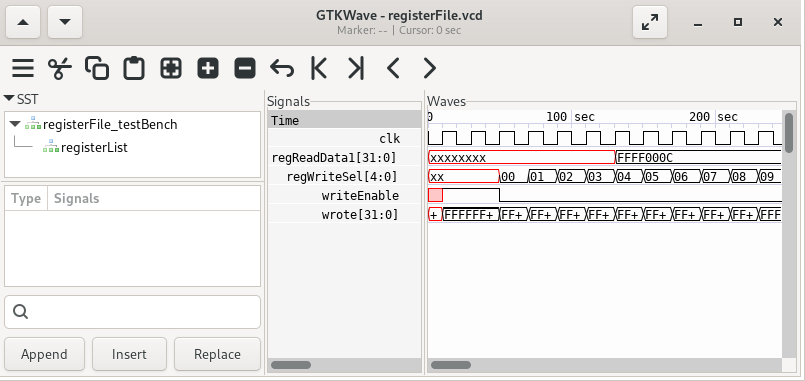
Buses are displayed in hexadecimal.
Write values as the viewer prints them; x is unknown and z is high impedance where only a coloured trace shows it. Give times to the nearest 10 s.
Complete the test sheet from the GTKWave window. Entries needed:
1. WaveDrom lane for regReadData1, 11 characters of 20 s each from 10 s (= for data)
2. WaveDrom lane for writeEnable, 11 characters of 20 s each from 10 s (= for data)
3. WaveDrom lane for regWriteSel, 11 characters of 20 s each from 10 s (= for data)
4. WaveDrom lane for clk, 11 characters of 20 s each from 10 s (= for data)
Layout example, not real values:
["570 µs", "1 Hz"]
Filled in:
["{name: 'regReadData1', wave: 'x.....=....', data: 'FFFF000C'}", "{name: 'writeEnable', wave: '1.0........'}", "{name: 'regWriteSel', wave: 'x.=========', data: '00 01 02 03 04 05 06 07 08'}", "{name: 'clk', wave: 'p..........'}"]
